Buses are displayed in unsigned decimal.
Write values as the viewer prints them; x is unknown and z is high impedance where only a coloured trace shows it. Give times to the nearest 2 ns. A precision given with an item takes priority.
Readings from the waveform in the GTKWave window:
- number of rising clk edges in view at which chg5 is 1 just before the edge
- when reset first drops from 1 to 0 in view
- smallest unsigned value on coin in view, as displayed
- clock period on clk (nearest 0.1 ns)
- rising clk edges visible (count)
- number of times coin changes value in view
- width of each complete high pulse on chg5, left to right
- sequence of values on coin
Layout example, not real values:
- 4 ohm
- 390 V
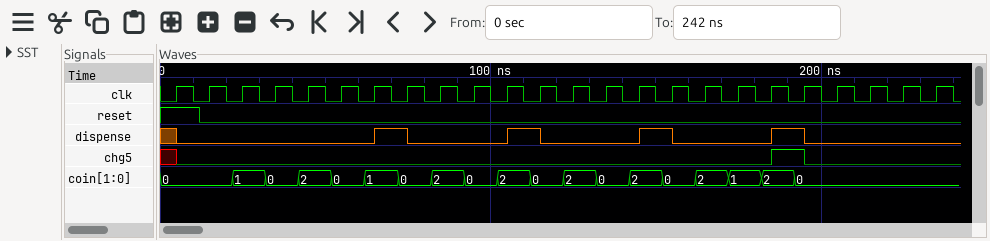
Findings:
- 1
- 12 ns
- 0
- 10 ns
- 24
- 18
- 10 ns
- 0, 1, 0, 2, 0, 1, 0, 2, 0, 2, 0, 2, 0, 2, 0, 2, 1, 2, 0
